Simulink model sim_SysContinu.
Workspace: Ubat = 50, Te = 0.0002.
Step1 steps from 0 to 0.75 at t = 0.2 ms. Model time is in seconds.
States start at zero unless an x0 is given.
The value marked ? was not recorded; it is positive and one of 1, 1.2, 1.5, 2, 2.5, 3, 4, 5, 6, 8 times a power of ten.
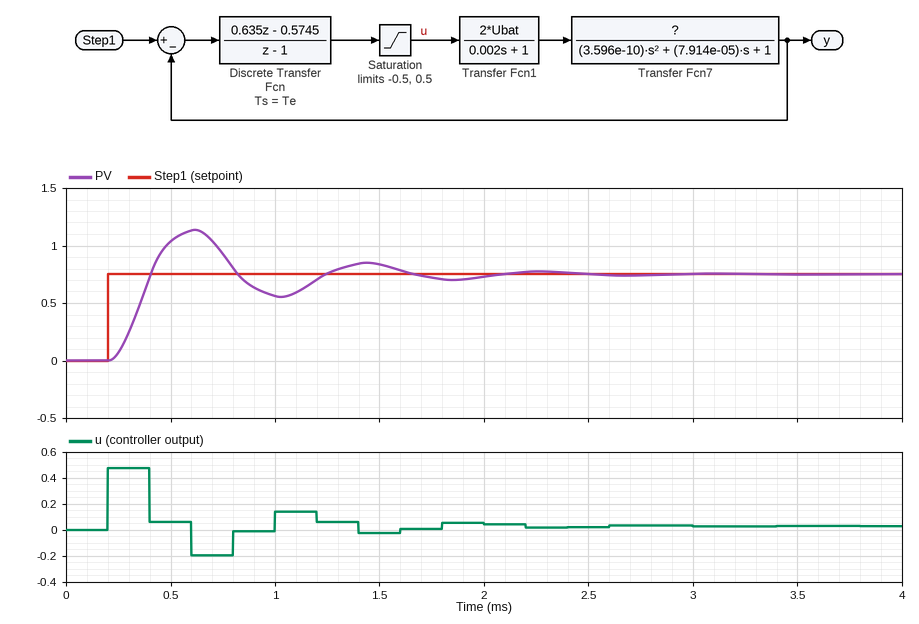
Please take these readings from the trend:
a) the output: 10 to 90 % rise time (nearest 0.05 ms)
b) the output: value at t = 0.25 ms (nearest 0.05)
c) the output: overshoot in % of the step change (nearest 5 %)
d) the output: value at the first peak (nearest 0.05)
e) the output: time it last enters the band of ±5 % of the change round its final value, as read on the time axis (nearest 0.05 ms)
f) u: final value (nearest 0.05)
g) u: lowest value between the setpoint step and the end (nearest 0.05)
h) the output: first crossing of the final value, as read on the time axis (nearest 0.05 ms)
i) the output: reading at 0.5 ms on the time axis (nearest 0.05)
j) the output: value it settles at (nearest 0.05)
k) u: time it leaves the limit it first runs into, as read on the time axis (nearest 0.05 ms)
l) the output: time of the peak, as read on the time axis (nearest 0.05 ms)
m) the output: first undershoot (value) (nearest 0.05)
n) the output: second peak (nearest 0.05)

0.15 ms
0.05
50 %
1.15
1.95 ms
0.05
-0.20
0.40 ms
1.05
0.75
0.40 ms
0.60 ms
0.55
0.85
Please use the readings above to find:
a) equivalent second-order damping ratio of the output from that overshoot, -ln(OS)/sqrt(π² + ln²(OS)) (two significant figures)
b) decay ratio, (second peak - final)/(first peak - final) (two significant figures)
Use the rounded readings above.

0.22
0.25
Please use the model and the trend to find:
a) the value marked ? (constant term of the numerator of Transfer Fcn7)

0.25
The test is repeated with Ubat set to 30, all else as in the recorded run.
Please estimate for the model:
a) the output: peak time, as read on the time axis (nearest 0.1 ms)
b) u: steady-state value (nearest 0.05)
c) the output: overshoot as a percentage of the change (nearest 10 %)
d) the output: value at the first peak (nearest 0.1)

0.7 ms
0.05
20 %
0.9
